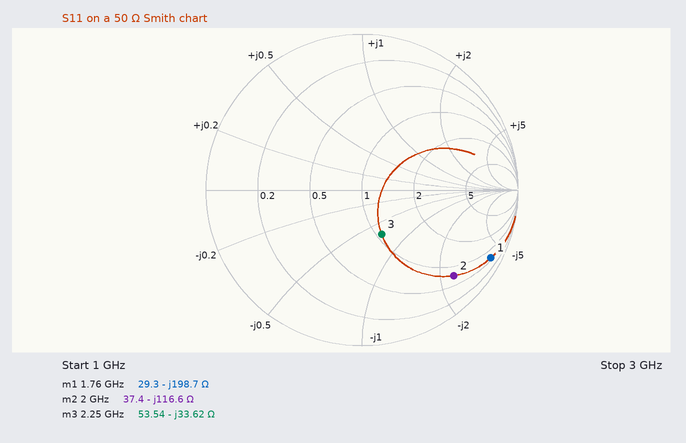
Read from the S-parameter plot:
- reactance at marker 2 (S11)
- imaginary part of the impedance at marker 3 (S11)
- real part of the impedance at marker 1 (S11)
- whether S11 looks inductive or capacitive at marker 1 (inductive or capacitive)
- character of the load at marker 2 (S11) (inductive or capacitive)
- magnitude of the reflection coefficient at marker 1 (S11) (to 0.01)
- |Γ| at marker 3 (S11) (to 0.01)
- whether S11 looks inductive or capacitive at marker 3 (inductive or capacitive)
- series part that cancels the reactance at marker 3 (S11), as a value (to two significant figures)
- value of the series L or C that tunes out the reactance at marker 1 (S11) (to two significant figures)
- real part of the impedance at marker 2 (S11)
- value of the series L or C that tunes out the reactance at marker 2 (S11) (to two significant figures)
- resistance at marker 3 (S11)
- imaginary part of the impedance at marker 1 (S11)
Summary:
-116.6 Ω
-33.62 Ω
29.3 Ω
capacitive
capacitive
0.93
0.31
capacitive
2.4 nH
18 nH
37.4 Ω
9.3 nH
53.54 Ω
-198.7 Ω
